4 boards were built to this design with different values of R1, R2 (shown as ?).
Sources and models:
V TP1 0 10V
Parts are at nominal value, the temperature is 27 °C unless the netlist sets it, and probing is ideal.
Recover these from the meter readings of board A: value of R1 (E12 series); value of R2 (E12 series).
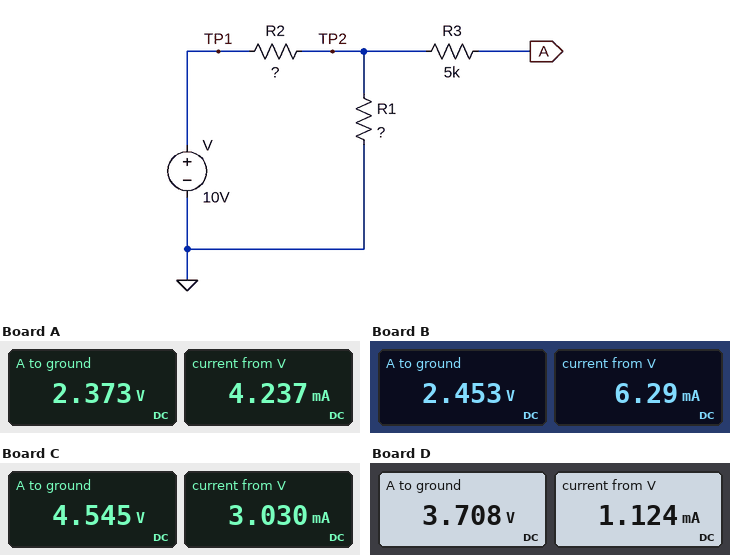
560 Ω
1.8 kΩ
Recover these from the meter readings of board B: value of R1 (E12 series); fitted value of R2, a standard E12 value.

390 Ω
1.2 kΩ
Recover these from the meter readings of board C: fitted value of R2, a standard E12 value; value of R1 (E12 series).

1.8 kΩ
1.5 kΩ
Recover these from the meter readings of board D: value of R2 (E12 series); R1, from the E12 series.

5.6 kΩ
3.3 kΩ
